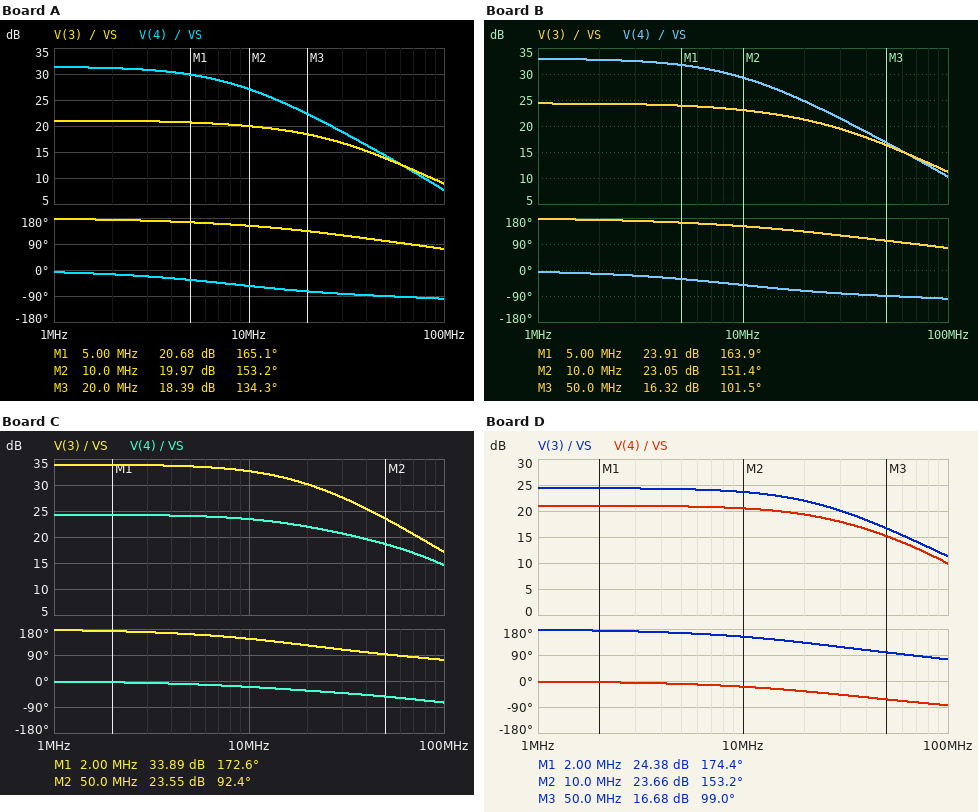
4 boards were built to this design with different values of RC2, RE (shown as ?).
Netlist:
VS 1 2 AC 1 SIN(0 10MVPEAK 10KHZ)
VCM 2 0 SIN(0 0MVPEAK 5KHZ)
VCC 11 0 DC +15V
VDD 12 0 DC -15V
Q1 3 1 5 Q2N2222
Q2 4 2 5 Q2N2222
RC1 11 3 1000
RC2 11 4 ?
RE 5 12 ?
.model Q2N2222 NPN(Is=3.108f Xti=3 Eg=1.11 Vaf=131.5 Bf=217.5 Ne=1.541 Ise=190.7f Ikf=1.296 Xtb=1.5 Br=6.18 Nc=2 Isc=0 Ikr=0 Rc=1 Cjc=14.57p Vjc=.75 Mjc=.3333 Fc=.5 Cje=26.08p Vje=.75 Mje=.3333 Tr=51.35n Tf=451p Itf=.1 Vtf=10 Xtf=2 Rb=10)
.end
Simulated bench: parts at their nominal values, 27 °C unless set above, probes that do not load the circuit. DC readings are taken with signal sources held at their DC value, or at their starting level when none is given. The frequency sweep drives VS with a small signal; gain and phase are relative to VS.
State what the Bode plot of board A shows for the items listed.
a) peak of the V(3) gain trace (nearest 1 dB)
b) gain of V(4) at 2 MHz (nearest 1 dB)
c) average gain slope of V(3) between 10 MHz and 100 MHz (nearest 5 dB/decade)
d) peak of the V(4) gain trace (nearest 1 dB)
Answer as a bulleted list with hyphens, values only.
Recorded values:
- 21 dB
- 31 dB
- -10 dB/decade
- 31 dB
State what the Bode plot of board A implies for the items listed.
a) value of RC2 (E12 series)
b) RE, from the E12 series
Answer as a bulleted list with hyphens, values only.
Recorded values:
- 3.3 kΩ
- 12 kΩ
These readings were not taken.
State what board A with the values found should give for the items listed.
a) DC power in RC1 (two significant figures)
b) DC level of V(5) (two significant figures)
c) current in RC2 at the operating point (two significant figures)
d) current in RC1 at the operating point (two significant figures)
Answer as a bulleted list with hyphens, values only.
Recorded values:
- 350 µW
- -670 mV
- 590 µA
- 590 µA
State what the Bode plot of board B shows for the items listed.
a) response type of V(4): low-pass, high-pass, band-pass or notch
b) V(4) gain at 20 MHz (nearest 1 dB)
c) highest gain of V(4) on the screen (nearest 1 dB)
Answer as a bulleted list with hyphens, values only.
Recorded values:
- low-pass
- 25 dB
- 33 dB
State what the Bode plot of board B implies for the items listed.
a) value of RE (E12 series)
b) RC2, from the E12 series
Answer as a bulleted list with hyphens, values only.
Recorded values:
- 8.2 kΩ
- 2.7 kΩ
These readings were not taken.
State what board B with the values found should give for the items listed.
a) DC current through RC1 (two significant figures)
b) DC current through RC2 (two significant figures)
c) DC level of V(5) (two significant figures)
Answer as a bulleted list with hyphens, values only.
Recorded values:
- 870 µA
- 860 µA
- -680 mV
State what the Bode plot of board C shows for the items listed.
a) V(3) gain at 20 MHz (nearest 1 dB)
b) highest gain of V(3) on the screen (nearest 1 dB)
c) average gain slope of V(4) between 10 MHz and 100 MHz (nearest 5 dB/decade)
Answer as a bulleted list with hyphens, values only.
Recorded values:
- 30 dB
- 34 dB
- -10 dB/decade
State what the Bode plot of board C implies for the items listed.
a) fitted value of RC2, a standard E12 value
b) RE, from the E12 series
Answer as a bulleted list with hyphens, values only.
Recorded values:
- 330 Ω
- 2.7 kΩ
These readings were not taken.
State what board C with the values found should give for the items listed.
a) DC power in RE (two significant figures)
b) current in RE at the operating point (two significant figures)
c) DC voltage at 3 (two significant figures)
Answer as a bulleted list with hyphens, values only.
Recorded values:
- 76 mW
- 5.3 mA
- 12 V
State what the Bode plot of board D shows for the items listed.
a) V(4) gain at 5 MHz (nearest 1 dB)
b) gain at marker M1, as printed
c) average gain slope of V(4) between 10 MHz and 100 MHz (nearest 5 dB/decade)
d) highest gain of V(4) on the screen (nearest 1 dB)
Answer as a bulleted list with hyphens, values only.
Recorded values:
- 21 dB
- 24.38 dB
- -10 dB/decade
- 21 dB
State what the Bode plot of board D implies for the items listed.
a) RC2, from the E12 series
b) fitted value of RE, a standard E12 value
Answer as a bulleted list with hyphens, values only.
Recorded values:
- 680 Ω
- 8.2 kΩ
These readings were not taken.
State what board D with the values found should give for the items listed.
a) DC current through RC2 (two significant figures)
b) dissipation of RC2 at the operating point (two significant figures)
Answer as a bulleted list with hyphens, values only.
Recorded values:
- 870 µA
- 510 µW
